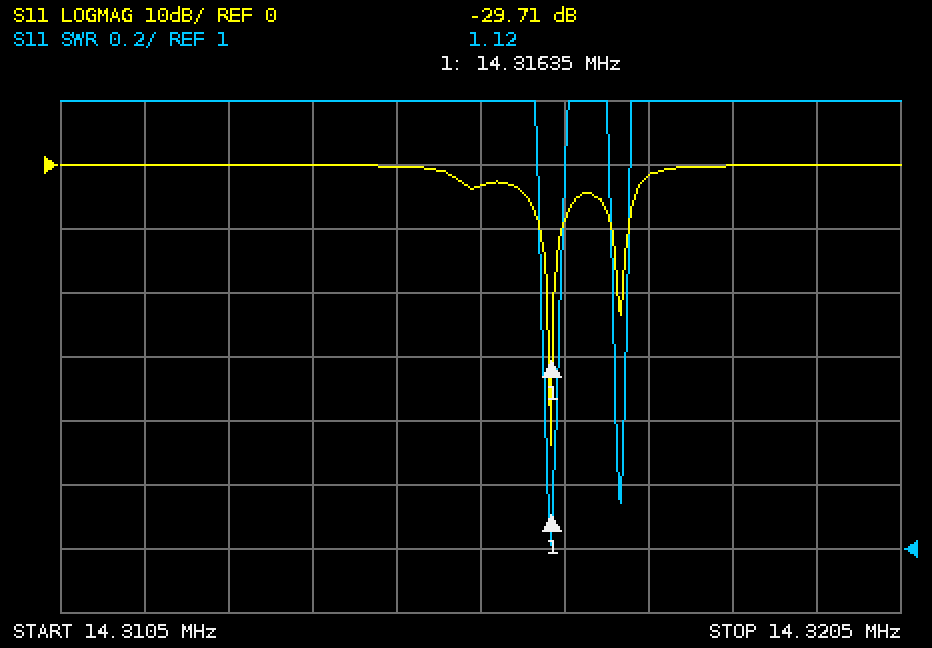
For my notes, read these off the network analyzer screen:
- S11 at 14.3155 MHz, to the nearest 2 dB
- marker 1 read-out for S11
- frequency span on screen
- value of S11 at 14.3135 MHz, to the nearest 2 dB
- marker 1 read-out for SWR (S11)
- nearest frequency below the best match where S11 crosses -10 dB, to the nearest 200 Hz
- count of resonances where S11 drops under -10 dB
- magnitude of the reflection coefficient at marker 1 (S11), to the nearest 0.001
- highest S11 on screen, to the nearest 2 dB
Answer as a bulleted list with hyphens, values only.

- -4 dB
- -29.71 dB
- 10 kHz
- 0 dB
- 1.12
- 14.3162 MHz
- 2
- 0.033
- 0 dB
